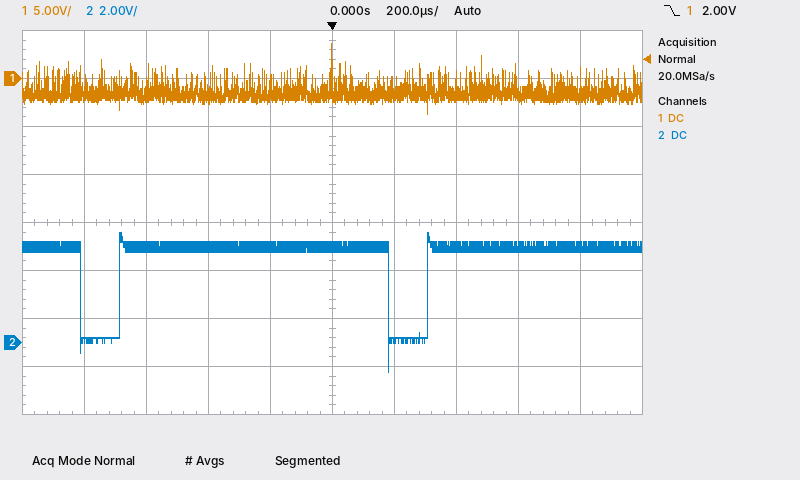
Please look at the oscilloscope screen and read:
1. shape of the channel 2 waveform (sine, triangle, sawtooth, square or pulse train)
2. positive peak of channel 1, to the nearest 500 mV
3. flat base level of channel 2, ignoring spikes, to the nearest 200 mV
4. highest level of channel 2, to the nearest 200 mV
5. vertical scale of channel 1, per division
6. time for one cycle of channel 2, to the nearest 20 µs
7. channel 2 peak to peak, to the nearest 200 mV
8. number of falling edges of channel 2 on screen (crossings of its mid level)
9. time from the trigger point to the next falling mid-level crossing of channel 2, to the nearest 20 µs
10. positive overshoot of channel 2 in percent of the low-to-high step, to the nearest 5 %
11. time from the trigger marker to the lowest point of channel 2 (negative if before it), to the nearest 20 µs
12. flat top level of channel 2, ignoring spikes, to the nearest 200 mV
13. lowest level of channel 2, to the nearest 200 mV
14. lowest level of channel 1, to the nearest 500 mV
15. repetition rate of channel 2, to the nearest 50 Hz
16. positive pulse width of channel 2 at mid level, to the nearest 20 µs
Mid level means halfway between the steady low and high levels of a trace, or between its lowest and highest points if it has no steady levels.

pulse train
3.5 V
200 mV
4.6 V
5 V
1.00 ms
5.8 V
2
180 µs
15 %
+180 µs
4.0 V
-1.2 V
-3.5 V
1.00 kHz
860 µs
